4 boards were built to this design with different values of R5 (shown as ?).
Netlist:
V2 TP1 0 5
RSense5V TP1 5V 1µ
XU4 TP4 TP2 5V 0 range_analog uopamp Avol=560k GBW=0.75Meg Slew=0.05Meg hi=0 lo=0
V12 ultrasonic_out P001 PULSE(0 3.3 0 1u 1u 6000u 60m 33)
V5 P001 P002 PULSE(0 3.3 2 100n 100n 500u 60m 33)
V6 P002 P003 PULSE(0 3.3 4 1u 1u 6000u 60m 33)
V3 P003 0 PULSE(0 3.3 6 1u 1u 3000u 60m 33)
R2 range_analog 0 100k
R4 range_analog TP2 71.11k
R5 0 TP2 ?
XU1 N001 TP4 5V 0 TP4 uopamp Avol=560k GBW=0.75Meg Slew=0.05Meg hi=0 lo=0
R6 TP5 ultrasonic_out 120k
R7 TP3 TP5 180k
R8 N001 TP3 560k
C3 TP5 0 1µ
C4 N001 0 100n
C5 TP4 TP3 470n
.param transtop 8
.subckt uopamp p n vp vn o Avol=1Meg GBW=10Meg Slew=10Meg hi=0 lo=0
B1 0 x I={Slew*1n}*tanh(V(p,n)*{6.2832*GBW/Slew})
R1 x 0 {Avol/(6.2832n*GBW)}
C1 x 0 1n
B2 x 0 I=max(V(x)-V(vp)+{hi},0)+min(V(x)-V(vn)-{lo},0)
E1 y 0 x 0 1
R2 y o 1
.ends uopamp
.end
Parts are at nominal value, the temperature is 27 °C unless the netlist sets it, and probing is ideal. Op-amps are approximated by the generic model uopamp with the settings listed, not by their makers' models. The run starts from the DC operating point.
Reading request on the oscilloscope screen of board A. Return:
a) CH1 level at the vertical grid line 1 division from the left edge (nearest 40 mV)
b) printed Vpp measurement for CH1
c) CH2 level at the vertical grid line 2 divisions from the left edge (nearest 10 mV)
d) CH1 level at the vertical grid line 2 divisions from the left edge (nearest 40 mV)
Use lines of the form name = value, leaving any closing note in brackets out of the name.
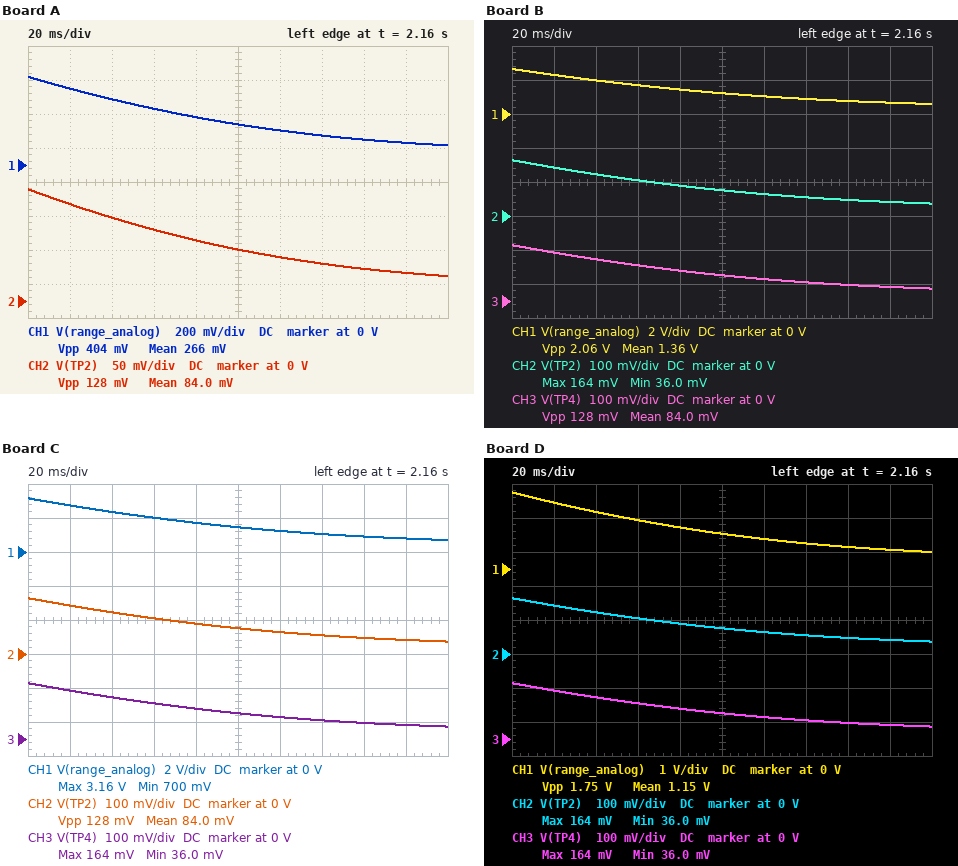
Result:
CH1 level at the vertical grid line 1 division from the left edge = 440 mV
printed Vpp measurement for CH1 = 404 mV
CH2 level at the vertical grid line 2 divisions from the left edge = 120 mV
CH1 level at the vertical grid line 2 divisions from the left edge = 400 mV
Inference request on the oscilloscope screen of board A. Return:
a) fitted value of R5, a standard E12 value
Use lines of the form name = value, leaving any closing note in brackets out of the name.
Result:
fitted value of R5, a standard E12 value = 33 kΩ
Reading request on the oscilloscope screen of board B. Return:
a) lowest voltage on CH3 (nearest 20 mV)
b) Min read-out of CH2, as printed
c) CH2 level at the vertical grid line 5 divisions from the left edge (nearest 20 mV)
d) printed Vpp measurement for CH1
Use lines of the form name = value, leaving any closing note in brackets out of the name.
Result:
lowest voltage on CH3 = 40 mV
Min read-out of CH2, as printed = 36.0 mV
CH2 level at the vertical grid line 5 divisions from the left edge = 80 mV
printed Vpp measurement for CH1 = 2.06 V
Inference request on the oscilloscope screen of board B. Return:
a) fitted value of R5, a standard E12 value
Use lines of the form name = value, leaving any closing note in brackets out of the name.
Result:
fitted value of R5, a standard E12 value = 4.7 kΩ
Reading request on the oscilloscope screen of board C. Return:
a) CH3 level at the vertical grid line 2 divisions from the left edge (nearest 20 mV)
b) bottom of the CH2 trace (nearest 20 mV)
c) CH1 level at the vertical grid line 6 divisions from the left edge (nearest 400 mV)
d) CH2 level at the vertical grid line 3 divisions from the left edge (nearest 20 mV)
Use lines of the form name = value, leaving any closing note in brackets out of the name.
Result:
CH3 level at the vertical grid line 2 divisions from the left edge = 120 mV
bottom of the CH2 trace = 40 mV
CH1 level at the vertical grid line 6 divisions from the left edge = 1.2 V
CH2 level at the vertical grid line 3 divisions from the left edge = 100 mV
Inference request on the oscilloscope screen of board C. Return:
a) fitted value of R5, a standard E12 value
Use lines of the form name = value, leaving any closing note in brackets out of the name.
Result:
fitted value of R5, a standard E12 value = 3.9 kΩ
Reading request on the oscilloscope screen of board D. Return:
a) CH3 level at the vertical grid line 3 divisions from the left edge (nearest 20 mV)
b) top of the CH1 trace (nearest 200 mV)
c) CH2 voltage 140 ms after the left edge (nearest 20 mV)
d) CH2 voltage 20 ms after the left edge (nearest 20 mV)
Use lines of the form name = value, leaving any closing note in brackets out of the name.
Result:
CH3 level at the vertical grid line 3 divisions from the left edge = 100 mV
top of the CH1 trace = 2.2 V
CH2 voltage 140 ms after the left edge = 60 mV
CH2 voltage 20 ms after the left edge = 140 mV
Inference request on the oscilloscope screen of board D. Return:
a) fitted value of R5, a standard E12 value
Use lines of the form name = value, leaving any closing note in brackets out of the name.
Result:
fitted value of R5, a standard E12 value = 5.6 kΩ
